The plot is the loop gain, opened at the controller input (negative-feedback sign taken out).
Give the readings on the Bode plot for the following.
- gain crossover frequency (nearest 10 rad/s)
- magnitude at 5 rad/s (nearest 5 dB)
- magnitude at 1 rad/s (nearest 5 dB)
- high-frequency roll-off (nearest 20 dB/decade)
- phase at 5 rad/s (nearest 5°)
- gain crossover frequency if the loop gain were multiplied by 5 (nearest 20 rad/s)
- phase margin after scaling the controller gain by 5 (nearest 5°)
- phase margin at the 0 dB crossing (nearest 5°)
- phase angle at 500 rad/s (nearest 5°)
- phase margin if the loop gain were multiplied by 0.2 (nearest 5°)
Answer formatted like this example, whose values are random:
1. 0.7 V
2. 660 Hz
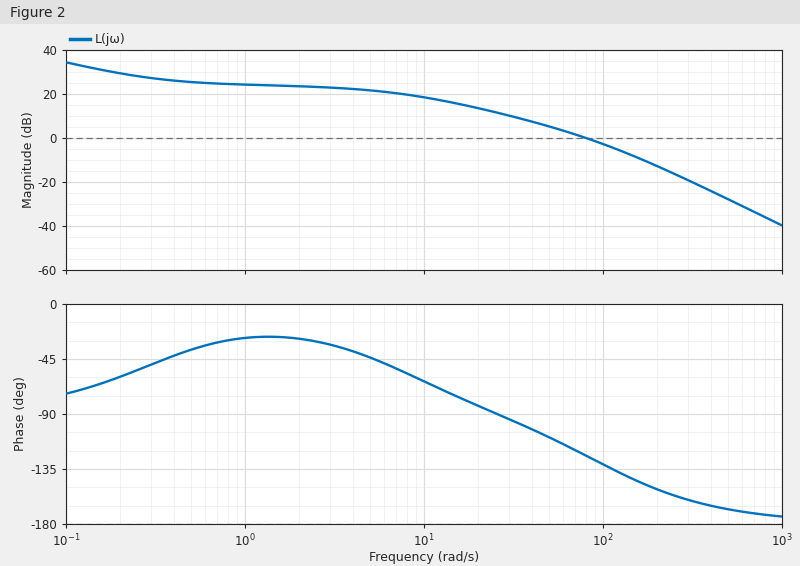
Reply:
1. 80 rad/s
2. 20 dB
3. 25 dB
4. -40 dB/decade
5. -45°
6. 220 rad/s
7. 25°
8. 55°
9. -170°
10. 100°
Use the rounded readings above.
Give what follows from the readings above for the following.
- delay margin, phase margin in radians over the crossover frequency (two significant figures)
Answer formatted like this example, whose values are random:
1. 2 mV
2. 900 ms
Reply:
1. 0.012 s
